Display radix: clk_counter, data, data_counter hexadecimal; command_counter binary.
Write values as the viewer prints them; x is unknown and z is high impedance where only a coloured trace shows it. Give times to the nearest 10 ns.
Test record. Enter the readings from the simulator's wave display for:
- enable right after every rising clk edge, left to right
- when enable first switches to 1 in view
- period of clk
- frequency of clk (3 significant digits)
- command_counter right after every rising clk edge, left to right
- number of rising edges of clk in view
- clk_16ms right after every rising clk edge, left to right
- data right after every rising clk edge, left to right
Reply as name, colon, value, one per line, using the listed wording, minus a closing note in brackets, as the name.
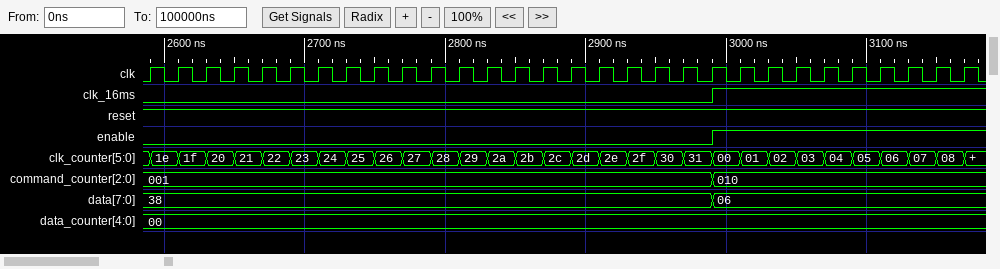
enable right after every rising clk edge, left to right: 0 0 0 0 0 0 0 0 0 0 0 0 0 0 0 0 0 0 0 0 1 1 1 1 1 1 1 1 1 1
when enable first switches to 1 in view: 2990 ns
period of clk: 20 ns
frequency of clk: 50.0 MHz
command_counter right after every rising clk edge, left to right: 001, 001, 001, 001, 001, 001, 001, 001, 001, 001, 001, 001, 001, 001, 001, 001, 001, 001, 001, 001, 010, 010, 010, 010, 010, 010, 010, 010, 010, 010
number of rising edges of clk in view: 30
clk_16ms right after every rising clk edge, left to right: 0 0 0 0 0 0 0 0 0 0 0 0 0 0 0 0 0 0 0 0 1 1 1 1 1 1 1 1 1 1
data right after every rising clk edge, left to right: 38, 38, 38, 38, 38, 38, 38, 38, 38, 38, 38, 38, 38, 38, 38, 38, 38, 38, 38, 38, 06, 06, 06, 06, 06, 06, 06, 06, 06, 06
